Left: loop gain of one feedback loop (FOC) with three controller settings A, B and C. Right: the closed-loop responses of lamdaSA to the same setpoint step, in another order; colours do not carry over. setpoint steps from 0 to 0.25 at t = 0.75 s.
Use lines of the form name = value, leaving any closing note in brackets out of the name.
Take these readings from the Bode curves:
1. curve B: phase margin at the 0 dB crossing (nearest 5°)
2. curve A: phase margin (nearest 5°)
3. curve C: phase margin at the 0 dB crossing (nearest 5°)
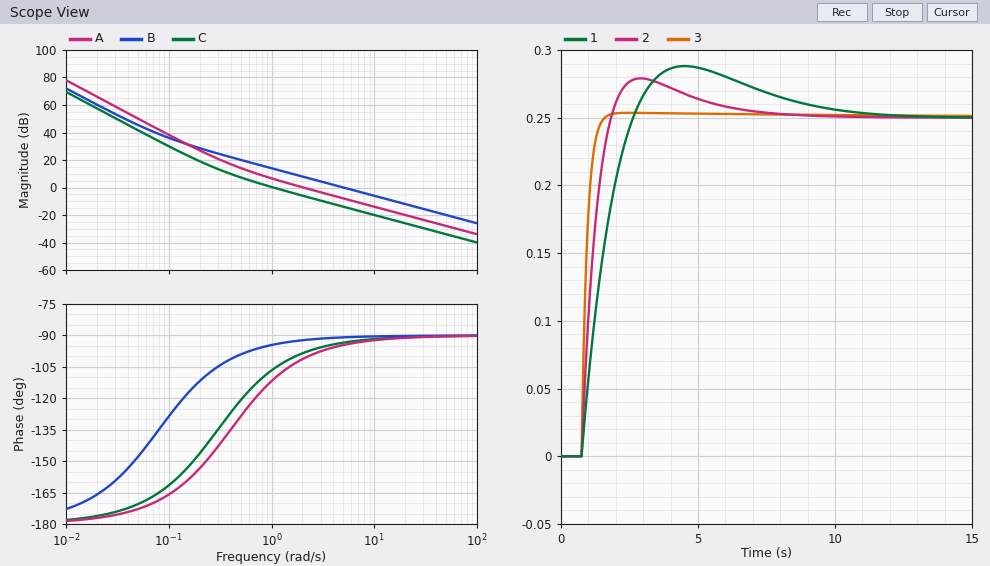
curve B: phase margin at the 0 dB crossing = 90°
curve A: phase margin = 80°
curve C: phase margin at the 0 dB crossing = 75°
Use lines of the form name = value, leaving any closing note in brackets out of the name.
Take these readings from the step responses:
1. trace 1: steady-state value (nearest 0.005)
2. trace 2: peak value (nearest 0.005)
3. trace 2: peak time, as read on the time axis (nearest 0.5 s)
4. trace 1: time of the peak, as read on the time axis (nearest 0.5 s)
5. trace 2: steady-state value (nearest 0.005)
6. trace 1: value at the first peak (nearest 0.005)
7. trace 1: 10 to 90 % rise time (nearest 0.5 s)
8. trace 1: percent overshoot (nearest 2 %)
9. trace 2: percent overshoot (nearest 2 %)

trace 1: steady-state value = 0.250
trace 2: peak value = 0.280
trace 2: peak time, as read on the time axis = 3.0 s
trace 1: time of the peak, as read on the time axis = 4.5 s
trace 2: steady-state value = 0.250
trace 1: value at the first peak = 0.290
trace 1: 10 to 90 % rise time = 1.5 s
trace 1: percent overshoot = 16 %
trace 2: percent overshoot = 12 %
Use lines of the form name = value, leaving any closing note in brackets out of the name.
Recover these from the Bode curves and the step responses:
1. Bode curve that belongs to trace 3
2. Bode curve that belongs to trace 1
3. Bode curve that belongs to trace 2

Bode curve that belongs to trace 3 = B
Bode curve that belongs to trace 1 = C
Bode curve that belongs to trace 2 = A
